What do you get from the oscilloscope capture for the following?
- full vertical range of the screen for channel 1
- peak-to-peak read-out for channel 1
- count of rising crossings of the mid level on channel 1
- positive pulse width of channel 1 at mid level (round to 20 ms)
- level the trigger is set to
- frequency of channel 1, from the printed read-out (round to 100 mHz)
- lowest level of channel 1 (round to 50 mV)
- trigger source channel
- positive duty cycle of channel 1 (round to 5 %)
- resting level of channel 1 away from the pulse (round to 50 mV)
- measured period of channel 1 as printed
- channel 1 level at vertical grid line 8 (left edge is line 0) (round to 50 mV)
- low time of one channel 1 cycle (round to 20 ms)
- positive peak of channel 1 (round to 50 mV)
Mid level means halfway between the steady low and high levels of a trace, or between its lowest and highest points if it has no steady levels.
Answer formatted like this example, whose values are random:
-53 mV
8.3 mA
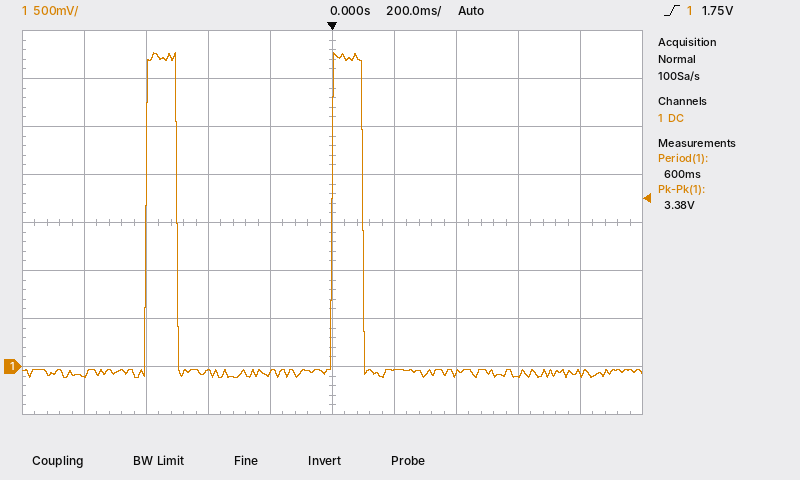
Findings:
4 V
3.38 V
2
100 ms
1.75 V
1.7 Hz
-100 mV
channel 1
15 %
-50 mV
600 ms
-100 mV
500 ms
3.25 V
